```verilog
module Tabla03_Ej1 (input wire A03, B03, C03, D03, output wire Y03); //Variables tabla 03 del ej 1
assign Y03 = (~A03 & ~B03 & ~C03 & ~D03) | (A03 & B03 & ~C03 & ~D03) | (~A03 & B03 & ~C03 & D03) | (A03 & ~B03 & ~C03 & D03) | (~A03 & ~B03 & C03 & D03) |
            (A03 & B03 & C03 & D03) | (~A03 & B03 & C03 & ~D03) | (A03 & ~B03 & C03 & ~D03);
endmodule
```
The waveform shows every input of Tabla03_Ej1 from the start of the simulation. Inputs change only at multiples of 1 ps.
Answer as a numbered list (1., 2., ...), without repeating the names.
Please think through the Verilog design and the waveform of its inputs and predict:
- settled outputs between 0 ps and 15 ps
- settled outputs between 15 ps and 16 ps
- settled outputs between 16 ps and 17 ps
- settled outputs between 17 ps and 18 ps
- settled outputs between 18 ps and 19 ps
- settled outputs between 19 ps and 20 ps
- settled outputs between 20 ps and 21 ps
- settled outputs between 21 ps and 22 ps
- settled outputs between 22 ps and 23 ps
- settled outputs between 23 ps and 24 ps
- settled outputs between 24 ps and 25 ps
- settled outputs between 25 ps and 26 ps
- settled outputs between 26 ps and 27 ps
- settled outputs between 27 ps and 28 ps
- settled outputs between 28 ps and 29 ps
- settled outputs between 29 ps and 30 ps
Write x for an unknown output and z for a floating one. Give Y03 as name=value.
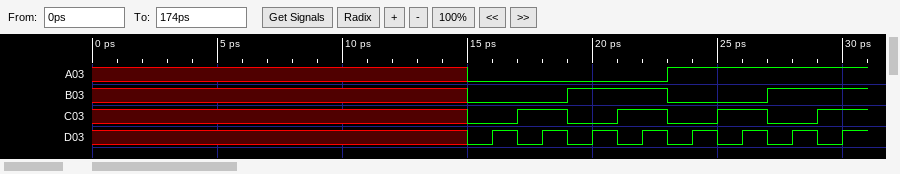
1. Y03=x
2. Y03=1
3. Y03=0
4. Y03=0
5. Y03=1
6. Y03=0
7. Y03=1
8. Y03=1
9. Y03=0
10. Y03=0
11. Y03=1
12. Y03=1
13. Y03=0
14. Y03=1
15. Y03=0
16. Y03=0
